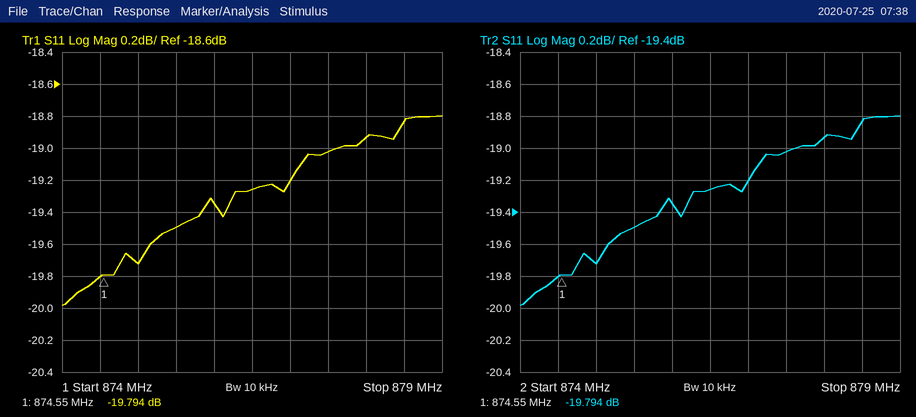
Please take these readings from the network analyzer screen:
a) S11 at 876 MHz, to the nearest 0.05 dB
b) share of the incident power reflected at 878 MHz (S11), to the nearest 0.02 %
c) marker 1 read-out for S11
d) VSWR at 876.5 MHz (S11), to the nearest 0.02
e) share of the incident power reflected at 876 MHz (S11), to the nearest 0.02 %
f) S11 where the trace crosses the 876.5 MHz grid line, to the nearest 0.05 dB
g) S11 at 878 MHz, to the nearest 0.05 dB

-19.35 dB
1.28 %
-19.794 dB
1.24
1.16 %
-19.25 dB
-18.95 dB
